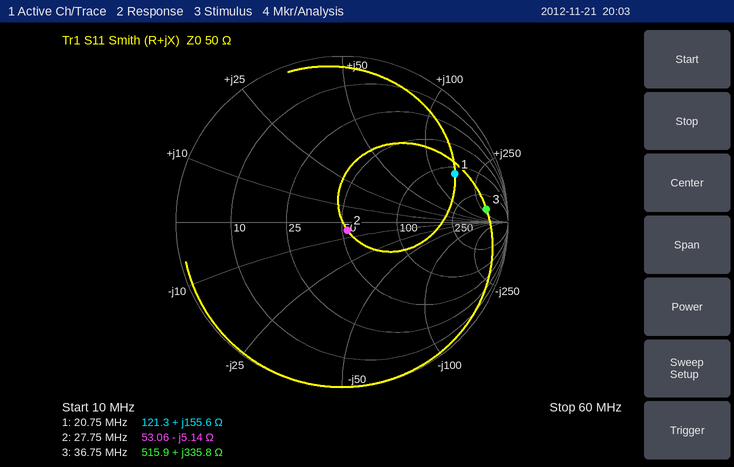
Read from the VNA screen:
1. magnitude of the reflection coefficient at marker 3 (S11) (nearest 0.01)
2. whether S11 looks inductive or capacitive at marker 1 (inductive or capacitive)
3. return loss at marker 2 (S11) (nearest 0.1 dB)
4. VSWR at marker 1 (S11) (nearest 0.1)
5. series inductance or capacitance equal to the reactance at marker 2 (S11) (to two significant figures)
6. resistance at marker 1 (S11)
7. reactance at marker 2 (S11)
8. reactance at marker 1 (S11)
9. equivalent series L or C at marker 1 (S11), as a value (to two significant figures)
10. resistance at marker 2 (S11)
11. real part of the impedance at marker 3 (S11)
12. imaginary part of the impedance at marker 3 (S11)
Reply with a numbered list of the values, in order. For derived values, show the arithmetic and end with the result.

1. 0.87
2. inductive
3. 24.7 dB
4. 6.7
5. C = 1/(2π × 27.75 MHz × 5.14 Ω) ≈ 1.1 nF
6. 121.3 Ω
7. -5.14 Ω
8. +155.6 Ω
9. L = 155.6 Ω/(2π × 20.75 MHz) ≈ 1.2 µH
10. 53.06 Ω
11. 515.9 Ω
12. +335.8 Ω
